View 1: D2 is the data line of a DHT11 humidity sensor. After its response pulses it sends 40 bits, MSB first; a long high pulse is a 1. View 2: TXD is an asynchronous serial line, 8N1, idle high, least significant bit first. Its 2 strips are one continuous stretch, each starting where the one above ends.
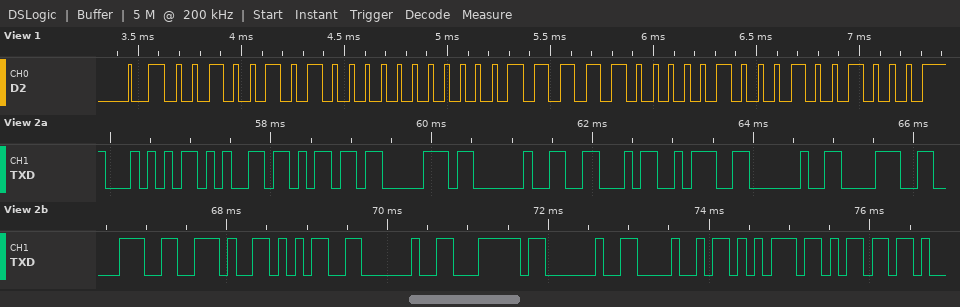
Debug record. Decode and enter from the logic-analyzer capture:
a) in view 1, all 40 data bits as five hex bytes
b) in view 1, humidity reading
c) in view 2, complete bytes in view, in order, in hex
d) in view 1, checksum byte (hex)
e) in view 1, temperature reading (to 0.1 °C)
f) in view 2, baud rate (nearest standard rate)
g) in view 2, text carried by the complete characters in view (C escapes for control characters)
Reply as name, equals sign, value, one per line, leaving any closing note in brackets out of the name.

in view 1, all 40 data bits as five hex bytes = 25 00 1F 04 48
in view 1, humidity reading = 37 %
in view 2, complete bytes in view, in order, in hex = 54 65 6D 70 20 46 3A 20 38 38 2E 35 20 7C 20 48 75 6D
in view 1, checksum byte = 0x48
in view 1, temperature reading = 31.4 °C
in view 2, baud rate = 9600 baud
in view 2, text carried by the complete characters in view = "Temp F: 88.5 | Hum"
